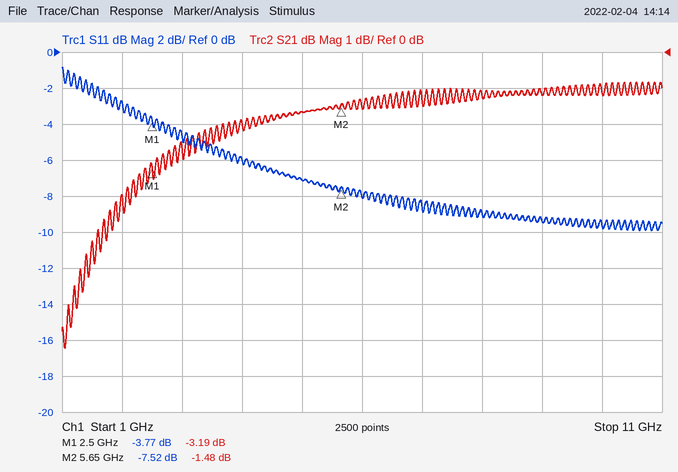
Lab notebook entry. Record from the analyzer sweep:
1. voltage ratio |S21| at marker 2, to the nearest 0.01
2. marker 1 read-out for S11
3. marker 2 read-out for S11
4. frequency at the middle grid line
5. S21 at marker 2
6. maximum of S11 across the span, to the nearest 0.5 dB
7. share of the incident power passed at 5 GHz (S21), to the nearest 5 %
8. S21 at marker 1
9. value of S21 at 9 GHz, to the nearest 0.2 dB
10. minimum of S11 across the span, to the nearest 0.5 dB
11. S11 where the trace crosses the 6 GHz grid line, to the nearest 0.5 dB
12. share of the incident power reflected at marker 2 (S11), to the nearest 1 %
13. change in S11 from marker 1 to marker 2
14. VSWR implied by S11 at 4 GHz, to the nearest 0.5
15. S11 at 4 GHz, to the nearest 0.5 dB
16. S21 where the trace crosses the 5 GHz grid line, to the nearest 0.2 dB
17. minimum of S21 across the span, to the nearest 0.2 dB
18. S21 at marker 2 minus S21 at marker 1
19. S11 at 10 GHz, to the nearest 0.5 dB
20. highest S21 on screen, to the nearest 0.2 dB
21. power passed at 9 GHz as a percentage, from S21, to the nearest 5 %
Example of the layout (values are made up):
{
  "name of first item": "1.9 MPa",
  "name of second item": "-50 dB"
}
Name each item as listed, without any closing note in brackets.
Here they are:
{
  "voltage ratio |S21| at marker 2, to the nearest 0.01": "0.84",
  "marker 1 read-out for S11": "-3.77 dB",
  "marker 2 read-out for S11": "-7.52 dB",
  "frequency at the middle grid line": "6 GHz",
  "S21 at marker 2": "-1.48 dB",
  "maximum of S11 across the span, to the nearest 0.5 dB": "-1.0 dB",
  "share of the incident power passed at 5 GHz (S21), to the nearest 5 %": "70 %",
  "S21 at marker 1": "-3.19 dB",
  "value of S21 at 9 GHz, to the nearest 0.2 dB": "-1.2 dB",
  "minimum of S11 across the span, to the nearest 0.5 dB": "-10.0 dB",
  "S11 where the trace crosses the 6 GHz grid line, to the nearest 0.5 dB": "-8.0 dB",
  "share of the incident power reflected at marker 2 (S11), to the nearest 1 %": "18 %",
  "change in S11 from marker 1 to marker 2": "-3.75 dB",
  "VSWR implied by S11 at 4 GHz, to the nearest 0.5": "3.0",
  "S11 at 4 GHz, to the nearest 0.5 dB": "-6.0 dB",
  "S21 where the trace crosses the 5 GHz grid line, to the nearest 0.2 dB": "-1.6 dB",
  "minimum of S21 across the span, to the nearest 0.2 dB": "-8.2 dB",
  "S21 at marker 2 minus S21 at marker 1": "1.71 dB",
  "S11 at 10 GHz, to the nearest 0.5 dB": "-9.5 dB",
  "highest S21 on screen, to the nearest 0.2 dB": "-0.8 dB",
  "power passed at 9 GHz as a percentage, from S21, to the nearest 5 %": "75 %"
}
